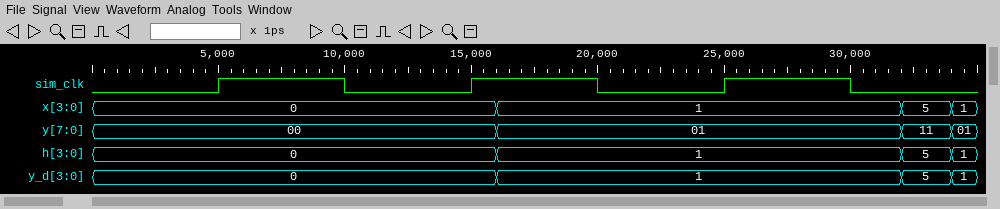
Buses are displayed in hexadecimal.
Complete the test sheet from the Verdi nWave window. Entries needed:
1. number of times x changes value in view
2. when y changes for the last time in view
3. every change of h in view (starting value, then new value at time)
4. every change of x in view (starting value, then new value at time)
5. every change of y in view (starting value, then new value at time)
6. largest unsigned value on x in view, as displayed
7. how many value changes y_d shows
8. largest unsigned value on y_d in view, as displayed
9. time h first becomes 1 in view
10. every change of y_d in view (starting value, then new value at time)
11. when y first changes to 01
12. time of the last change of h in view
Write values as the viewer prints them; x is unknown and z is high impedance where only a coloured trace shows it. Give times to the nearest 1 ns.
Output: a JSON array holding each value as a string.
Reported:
["3", "34 ns", "0, 1 at 16 ns, 5 at 32 ns, 1 at 34 ns", "0, 1 at 16 ns, 5 at 32 ns, 1 at 34 ns", "00, 01 at 16 ns, 11 at 32 ns, 01 at 34 ns", "5", "3", "5", "16 ns", "0, 1 at 16 ns, 5 at 32 ns, 1 at 34 ns", "16 ns", "34 ns"]
